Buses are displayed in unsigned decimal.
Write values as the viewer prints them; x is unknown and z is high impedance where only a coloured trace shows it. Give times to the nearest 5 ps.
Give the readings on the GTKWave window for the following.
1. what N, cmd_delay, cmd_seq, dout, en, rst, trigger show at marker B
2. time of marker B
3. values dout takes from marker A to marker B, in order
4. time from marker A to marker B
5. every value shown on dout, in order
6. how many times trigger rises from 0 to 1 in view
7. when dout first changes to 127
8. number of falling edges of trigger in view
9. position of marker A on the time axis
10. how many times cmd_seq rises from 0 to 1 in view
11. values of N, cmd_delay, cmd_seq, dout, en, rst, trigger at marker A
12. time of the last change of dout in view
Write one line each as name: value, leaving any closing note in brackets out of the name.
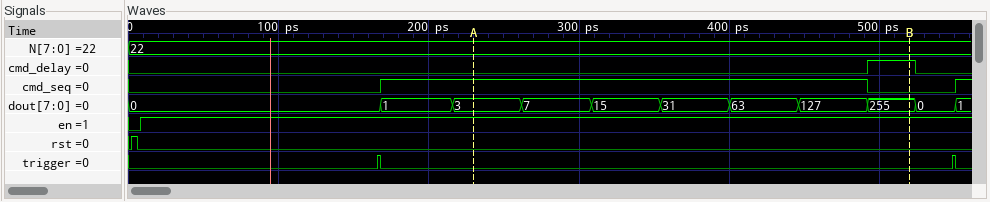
what N, cmd_delay, cmd_seq, dout, en, rst, trigger show at marker B: N=22, cmd_delay=1, cmd_seq=0, dout=255, en=1, rst=0, trigger=0
time of marker B: 520 ps
values dout takes from marker A to marker B, in order: 3, 7, 15, 31, 63, 127, 255
time from marker A to marker B: 290 ps
every value shown on dout, in order: 0, 1, 3, 7, 15, 31, 63, 127, 255, 0, 1
how many times trigger rises from 0 to 1 in view: 2
when dout first changes to 127: 445 ps
number of falling edges of trigger in view: 2
position of marker A on the time axis: 230 ps
how many times cmd_seq rises from 0 to 1 in view: 2
values of N, cmd_delay, cmd_seq, dout, en, rst, trigger at marker A: N=22, cmd_delay=0, cmd_seq=1, dout=3, en=1, rst=0, trigger=0
time of the last change of dout in view: 550 ps
